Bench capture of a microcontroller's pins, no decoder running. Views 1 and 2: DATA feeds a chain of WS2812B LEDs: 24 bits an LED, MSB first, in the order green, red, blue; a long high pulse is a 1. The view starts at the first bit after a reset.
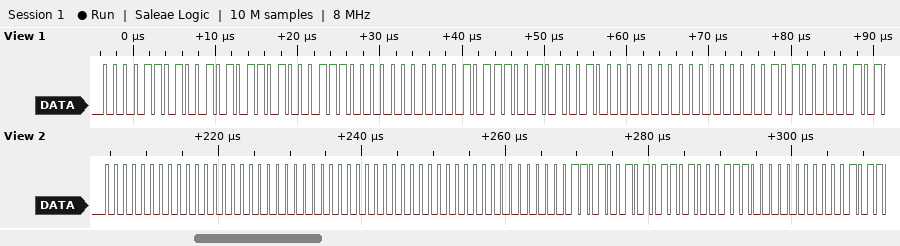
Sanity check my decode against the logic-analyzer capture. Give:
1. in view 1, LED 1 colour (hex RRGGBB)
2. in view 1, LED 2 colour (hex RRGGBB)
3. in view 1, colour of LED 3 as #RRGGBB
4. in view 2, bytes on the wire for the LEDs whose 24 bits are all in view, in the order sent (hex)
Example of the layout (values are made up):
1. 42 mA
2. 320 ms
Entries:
1. #2B0D47
2. #170029
3. #000050
4. 00 00 00 00 00 00 0D 2B 47
